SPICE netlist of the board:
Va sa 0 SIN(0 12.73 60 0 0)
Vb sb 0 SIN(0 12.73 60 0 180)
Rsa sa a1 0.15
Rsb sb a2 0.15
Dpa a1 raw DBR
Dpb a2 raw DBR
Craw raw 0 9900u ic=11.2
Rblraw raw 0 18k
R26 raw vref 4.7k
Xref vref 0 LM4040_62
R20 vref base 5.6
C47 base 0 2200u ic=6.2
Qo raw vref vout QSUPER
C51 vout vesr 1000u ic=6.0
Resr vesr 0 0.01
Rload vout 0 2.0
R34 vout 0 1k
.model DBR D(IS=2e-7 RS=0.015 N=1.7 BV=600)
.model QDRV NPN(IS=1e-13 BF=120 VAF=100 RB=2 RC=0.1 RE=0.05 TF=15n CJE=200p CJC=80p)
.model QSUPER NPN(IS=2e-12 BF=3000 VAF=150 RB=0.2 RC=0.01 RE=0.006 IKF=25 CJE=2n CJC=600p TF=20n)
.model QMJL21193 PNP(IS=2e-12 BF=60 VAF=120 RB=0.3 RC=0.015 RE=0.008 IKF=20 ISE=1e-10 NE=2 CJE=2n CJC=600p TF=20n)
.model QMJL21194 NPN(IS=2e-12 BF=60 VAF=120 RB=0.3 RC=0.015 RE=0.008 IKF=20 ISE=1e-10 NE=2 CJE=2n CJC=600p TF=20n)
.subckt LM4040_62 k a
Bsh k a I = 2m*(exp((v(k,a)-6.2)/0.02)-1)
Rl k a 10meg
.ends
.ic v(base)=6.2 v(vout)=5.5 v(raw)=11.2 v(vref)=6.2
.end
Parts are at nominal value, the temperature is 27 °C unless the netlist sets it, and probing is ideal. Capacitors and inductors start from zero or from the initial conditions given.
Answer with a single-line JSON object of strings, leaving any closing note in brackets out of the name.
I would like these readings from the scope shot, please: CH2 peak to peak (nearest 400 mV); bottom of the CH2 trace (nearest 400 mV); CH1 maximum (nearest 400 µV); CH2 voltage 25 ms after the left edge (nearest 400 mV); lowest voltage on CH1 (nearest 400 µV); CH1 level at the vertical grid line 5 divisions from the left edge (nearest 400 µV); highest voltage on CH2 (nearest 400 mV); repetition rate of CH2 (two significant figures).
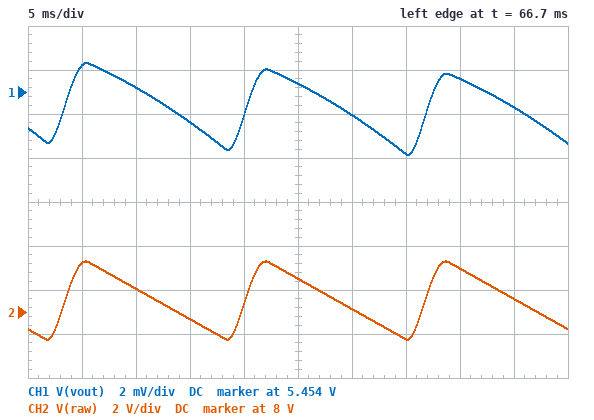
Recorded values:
{"CH2 peak to peak": "3.6 V", "bottom of the CH2 trace": "6.8 V", "CH1 maximum": "5.4552 V", "CH2 voltage 25 ms after the left edge": "9.6 V", "lowest voltage on CH1": "5.4512 V", "CH1 level at the vertical grid line 5 divisions from the left edge": "5.4544 V", "highest voltage on CH2": "10.4 V", "repetition rate of CH2": "60 Hz"}
